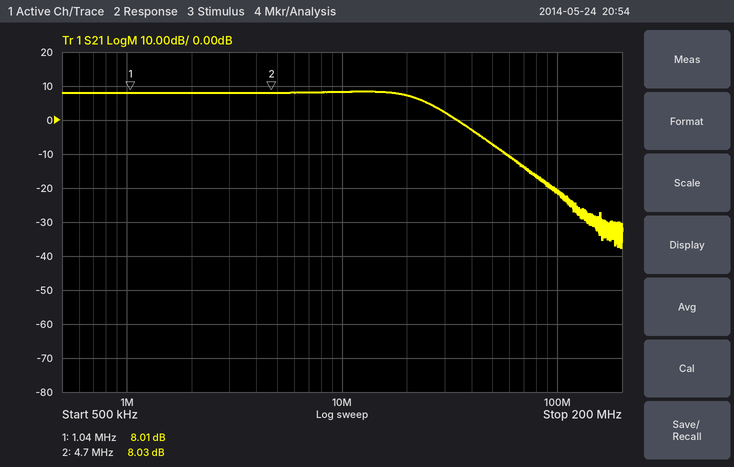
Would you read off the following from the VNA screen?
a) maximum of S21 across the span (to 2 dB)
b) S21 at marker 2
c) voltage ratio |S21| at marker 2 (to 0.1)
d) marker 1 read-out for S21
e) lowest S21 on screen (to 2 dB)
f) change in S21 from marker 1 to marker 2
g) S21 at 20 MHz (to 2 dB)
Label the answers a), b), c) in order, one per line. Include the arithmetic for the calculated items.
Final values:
a) 8 dB
b) 8.03 dB
c) 10^(8.03/20) ≈ 2.5
d) 8.01 dB
e) -38 dB
f) 8.03 − (8.01) = 0.02 dB
g) 8 dB
